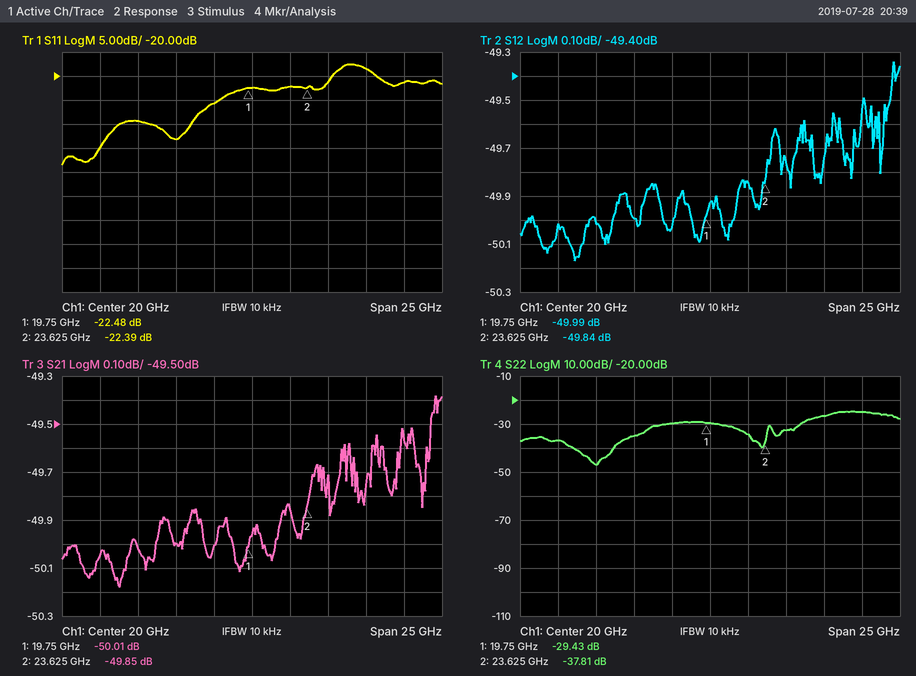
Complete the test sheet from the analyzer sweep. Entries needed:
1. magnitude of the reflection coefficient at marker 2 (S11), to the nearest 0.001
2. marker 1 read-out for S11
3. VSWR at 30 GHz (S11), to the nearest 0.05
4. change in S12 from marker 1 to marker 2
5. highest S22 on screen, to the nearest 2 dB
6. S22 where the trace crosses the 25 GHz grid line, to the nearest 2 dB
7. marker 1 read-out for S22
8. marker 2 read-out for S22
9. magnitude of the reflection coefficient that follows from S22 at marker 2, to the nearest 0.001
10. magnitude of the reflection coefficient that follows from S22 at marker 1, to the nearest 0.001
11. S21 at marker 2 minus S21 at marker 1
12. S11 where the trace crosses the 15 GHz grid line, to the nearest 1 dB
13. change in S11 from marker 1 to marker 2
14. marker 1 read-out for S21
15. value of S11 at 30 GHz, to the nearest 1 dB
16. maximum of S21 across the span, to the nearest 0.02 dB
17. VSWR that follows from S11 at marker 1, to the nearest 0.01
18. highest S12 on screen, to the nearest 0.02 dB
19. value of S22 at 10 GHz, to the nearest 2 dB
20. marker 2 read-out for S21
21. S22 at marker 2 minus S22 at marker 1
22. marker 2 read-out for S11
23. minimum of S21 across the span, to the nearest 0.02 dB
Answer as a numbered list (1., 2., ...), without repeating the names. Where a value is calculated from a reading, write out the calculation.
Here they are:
1. 10^(-22.39/20) ≈ 0.076
2. -22.48 dB
3. |Γ| = 10^(-21/20) = 0.0891; VSWR = (1 + 0.0891)/(1 − 0.0891) ≈ 1.20
4. -49.84 − (-49.99) = 0.15 dB
5. -24 dB
6. -32 dB
7. -29.43 dB
8. -37.81 dB
9. 10^(-37.81/20) ≈ 0.013
10. 10^(-29.43/20) ≈ 0.034
11. -49.85 − (-50.01) = 0.16 dB
12. -33 dB
13. -22.39 − (-22.48) = 0.09 dB
14. -50.01 dB
15. -21 dB
16. -49.38 dB
17. (1 + 0.0752)/(1 − 0.0752) ≈ 1.16
18. -49.34 dB
19. -36 dB
20. -49.85 dB
21. -37.81 − (-29.43) = -8.38 dB
22. -22.39 dB
23. -50.18 dB
